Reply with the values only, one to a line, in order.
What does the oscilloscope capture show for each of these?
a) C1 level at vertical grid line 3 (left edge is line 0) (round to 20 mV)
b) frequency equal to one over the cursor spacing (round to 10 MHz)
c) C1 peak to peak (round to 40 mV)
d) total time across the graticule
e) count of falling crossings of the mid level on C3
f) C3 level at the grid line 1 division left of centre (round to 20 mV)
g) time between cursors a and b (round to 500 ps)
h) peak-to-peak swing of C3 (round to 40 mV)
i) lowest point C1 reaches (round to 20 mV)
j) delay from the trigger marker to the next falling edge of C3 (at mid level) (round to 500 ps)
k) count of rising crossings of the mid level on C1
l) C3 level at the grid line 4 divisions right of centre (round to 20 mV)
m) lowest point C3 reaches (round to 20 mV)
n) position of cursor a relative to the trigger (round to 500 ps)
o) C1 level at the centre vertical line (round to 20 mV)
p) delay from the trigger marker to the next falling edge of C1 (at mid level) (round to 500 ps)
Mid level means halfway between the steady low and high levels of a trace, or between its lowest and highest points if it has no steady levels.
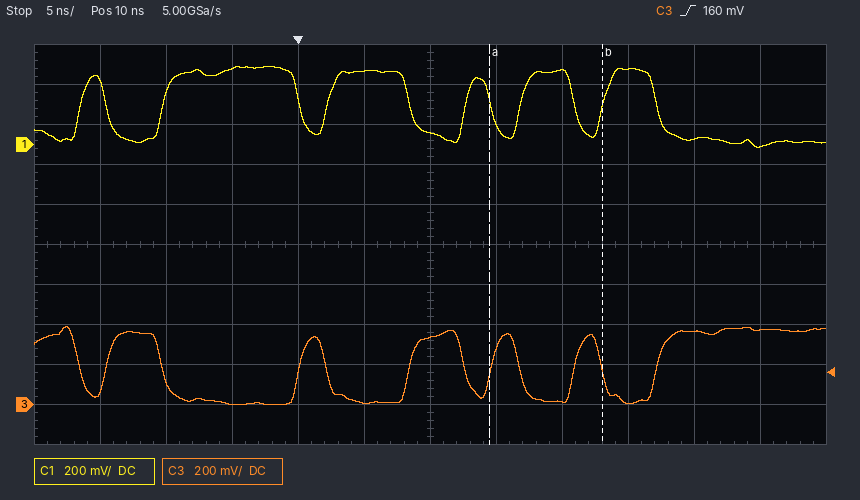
380 mV
120 MHz
400 mV
60 ns
6
0 mV
8.5 ns
400 mV
-20 mV
2.0 ns
6
360 mV
0 mV
+14.5 ns
60 mV
8.5 ns
